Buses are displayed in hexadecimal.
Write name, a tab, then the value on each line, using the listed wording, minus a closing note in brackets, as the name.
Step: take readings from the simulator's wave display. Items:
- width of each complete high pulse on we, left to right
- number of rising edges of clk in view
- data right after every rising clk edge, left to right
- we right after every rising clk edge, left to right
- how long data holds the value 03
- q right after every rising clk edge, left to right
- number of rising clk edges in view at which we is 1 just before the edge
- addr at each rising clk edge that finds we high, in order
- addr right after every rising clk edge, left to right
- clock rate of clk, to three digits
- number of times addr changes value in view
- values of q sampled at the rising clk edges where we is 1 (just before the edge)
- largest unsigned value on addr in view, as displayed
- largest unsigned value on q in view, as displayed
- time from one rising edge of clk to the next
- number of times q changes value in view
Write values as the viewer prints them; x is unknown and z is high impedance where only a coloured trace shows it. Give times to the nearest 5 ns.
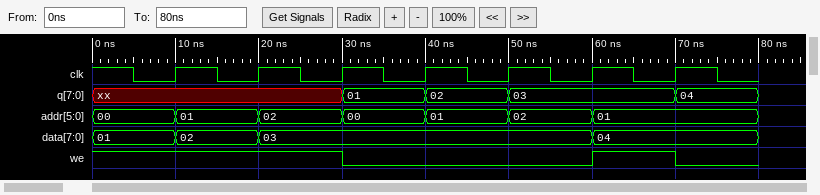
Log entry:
width of each complete high pulse on we, left to right	10 ns
number of rising edges of clk in view	7
data right after every rising clk edge, left to right	02, 03, 03, 03, 03, 04, 04
we right after every rising clk edge, left to right	1 1 0 0 0 1 0
how long data holds the value 03	40 ns
q right after every rising clk edge, left to right	xx, xx, 01, 02, 03, 03, 04
number of rising clk edges in view at which we is 1 just before the edge	4
addr at each rising clk edge that finds we high, in order	00, 01, 02, 01
addr right after every rising clk edge, left to right	01, 02, 00, 01, 02, 01, 01
clock rate of clk, to three digits	100 MHz
number of times addr changes value in view	6
values of q sampled at the rising clk edges where we is 1	xx, xx, xx, 03
largest unsigned value on addr in view, as displayed	02
largest unsigned value on q in view, as displayed	04
time from one rising edge of clk to the next	10 ns
number of times q changes value in view	4
